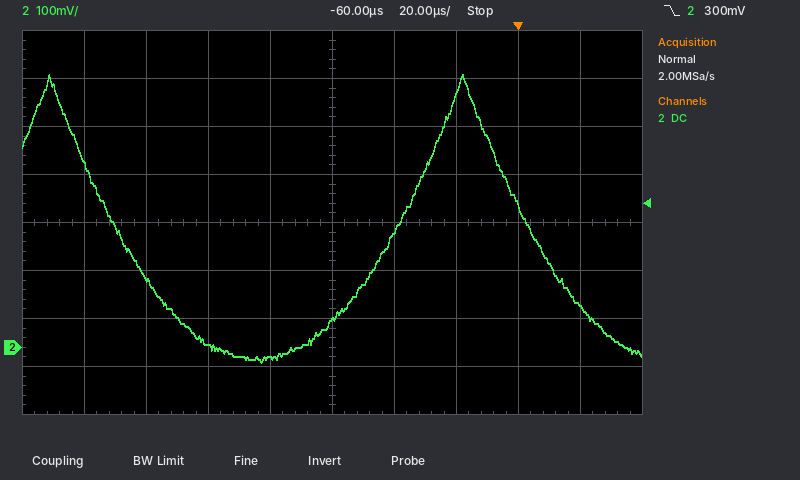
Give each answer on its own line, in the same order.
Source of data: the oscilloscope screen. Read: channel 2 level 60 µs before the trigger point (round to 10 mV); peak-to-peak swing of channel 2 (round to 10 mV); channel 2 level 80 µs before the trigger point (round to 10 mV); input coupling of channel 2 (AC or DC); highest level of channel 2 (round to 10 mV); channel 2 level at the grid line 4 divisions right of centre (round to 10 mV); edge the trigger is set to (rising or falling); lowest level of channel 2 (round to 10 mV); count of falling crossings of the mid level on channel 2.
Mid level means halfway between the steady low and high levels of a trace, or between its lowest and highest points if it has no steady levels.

60 mV
600 mV
-20 mV
DC
570 mV
90 mV
falling
-30 mV
2
